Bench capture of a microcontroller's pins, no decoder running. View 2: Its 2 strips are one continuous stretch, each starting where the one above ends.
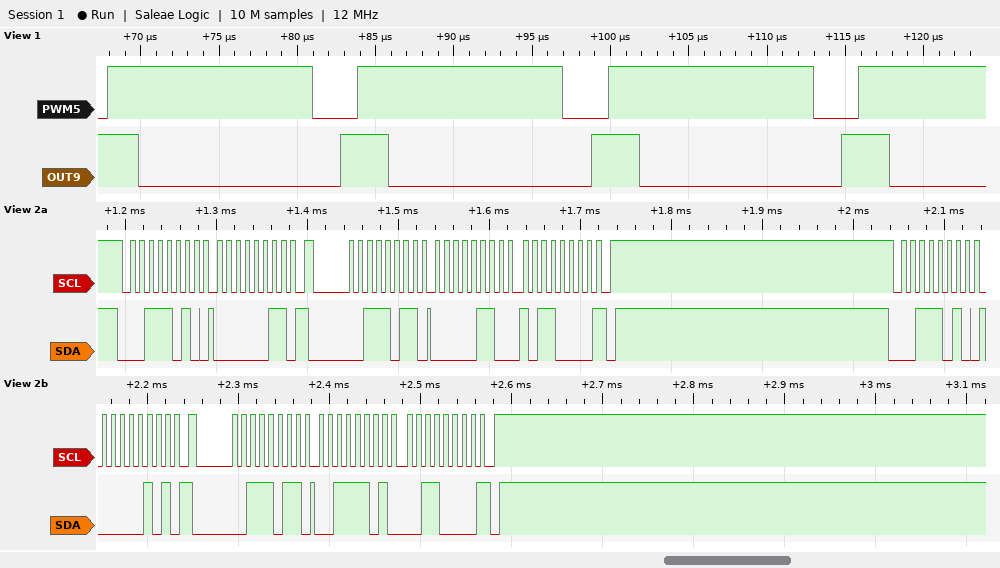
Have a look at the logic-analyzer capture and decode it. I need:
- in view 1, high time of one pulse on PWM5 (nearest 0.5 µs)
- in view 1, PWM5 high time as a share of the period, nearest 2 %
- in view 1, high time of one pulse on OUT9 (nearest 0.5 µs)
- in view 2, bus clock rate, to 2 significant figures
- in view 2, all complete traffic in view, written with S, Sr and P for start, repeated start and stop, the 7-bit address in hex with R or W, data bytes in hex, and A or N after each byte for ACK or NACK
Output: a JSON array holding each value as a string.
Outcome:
["13.0 µs", "82 %", "3.0 µs", "100 kHz", "S 1DW A 03 A Sr 1DR A 06 A B0 N P S 1DW A 05 A Sr 1DR A 3D A 30 N P"]
